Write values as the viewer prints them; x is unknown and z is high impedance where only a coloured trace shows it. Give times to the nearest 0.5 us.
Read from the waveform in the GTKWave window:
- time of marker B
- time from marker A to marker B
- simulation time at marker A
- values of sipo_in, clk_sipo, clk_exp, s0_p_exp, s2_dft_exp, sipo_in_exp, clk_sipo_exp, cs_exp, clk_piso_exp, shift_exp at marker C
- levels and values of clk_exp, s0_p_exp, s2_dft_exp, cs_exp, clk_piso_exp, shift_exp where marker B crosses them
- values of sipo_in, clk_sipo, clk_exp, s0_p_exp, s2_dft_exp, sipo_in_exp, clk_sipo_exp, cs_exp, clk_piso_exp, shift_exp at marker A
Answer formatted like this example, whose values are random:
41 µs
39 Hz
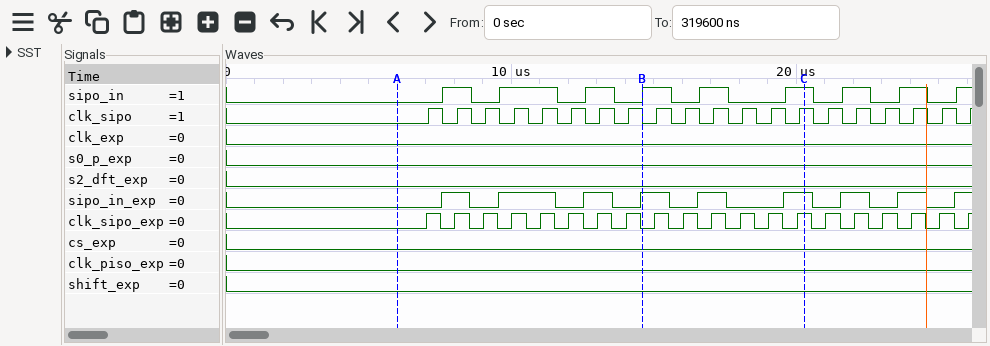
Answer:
14.5 us
8.5 us
6 us
sipo_in=1, clk_sipo=1, clk_exp=0, s0_p_exp=0, s2_dft_exp=0, sipo_in_exp=1, clk_sipo_exp=1, cs_exp=0, clk_piso_exp=0, shift_exp=0
clk_exp=0, s0_p_exp=0, s2_dft_exp=0, cs_exp=0, clk_piso_exp=0, shift_exp=0
sipo_in=0, clk_sipo=0, clk_exp=0, s0_p_exp=0, s2_dft_exp=0, sipo_in_exp=0, clk_sipo_exp=0, cs_exp=0, clk_piso_exp=0, shift_exp=0
